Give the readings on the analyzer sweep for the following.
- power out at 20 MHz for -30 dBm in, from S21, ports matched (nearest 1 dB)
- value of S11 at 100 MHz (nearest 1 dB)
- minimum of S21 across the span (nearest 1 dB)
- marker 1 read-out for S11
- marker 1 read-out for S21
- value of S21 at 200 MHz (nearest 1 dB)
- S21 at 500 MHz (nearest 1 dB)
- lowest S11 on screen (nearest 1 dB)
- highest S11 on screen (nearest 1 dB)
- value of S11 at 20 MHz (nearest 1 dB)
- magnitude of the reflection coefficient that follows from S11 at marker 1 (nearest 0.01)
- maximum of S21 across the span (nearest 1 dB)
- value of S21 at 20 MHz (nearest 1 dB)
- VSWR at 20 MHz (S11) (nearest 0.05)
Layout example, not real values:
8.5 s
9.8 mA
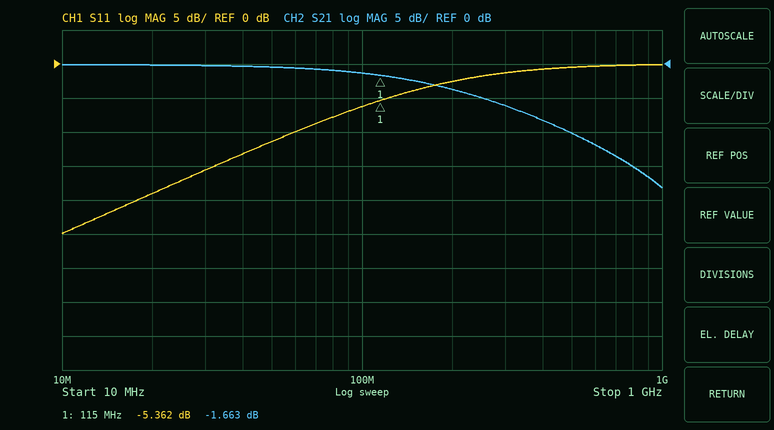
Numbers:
-30 dBm
-6 dB
-18 dB
-5.362 dB
-1.663 dB
-4 dB
-10 dB
-25 dB
0 dB
-19 dB
0.54
0 dB
0 dB
1.25
